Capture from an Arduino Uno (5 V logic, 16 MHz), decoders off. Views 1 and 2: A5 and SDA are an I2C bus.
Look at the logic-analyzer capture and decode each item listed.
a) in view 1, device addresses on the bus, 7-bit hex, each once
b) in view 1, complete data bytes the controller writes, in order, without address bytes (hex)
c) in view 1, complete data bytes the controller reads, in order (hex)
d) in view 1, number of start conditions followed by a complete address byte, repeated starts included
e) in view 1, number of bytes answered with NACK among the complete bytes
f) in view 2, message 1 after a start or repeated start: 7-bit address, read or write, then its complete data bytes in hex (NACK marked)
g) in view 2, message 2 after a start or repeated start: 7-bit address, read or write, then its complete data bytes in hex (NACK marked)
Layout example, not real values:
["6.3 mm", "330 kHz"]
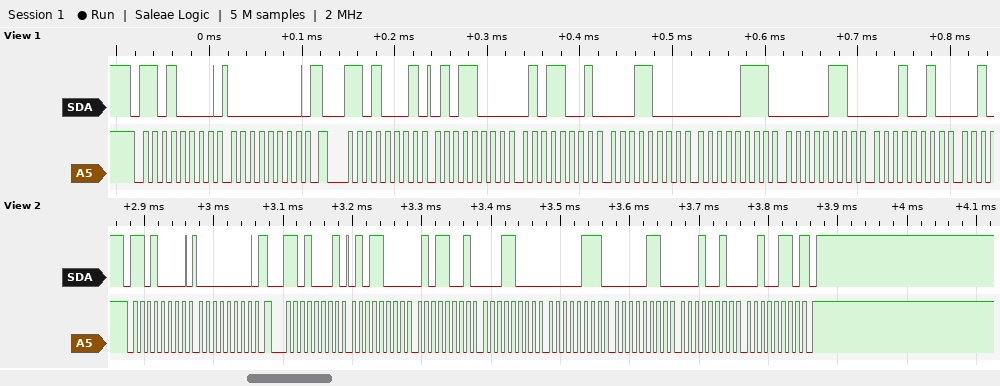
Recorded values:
["0x68", "00", "58 59 18 07 06 12", "2", "0", "0x68 write: 00", "0x68 read: 58 59 18 07 06 12 26 NACK"]
